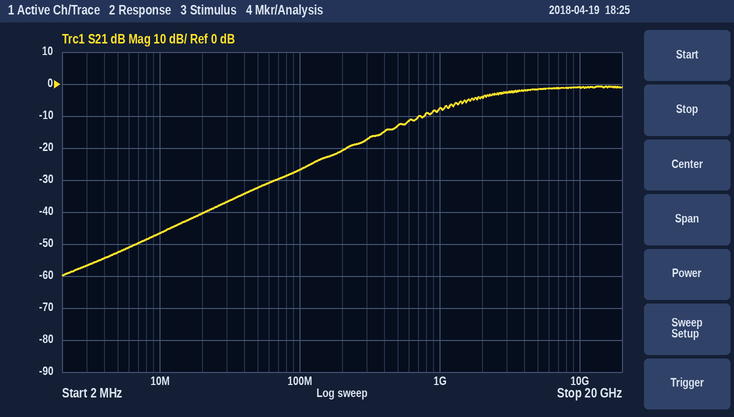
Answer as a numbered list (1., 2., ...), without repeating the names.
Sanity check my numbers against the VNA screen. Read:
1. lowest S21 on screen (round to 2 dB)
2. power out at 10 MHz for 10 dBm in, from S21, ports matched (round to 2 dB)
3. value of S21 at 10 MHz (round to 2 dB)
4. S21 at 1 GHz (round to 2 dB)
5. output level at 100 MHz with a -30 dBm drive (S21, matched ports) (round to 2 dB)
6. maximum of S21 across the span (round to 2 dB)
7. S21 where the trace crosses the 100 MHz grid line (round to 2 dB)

1. -60 dB
2. -36 dBm
3. -46 dB
4. -8 dB
5. -56 dBm
6. 0 dB
7. -26 dB
